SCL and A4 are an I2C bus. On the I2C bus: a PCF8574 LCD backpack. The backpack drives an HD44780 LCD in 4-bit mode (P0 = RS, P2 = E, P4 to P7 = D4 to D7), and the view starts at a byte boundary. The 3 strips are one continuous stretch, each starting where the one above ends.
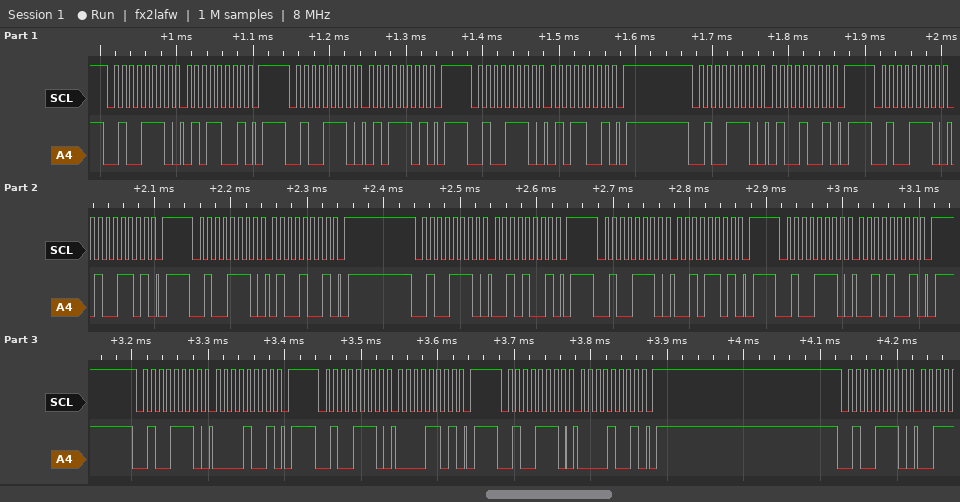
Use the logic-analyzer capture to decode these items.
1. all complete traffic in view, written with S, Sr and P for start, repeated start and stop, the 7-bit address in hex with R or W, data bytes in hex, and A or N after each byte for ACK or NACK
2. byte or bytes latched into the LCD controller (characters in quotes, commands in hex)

S 27W A 59 A P S 27W A 5D A P S 27W A 59 A P S 27W A 49 A P S 27W A 4D A P S 27W A 49 A P S 27W A 29 A P S 27W A 2D A P S 27W A 29 A P S 27W A 09 A P S 27W A 0D A P S 27W A 09 A P S 27W A
'T' ' '
